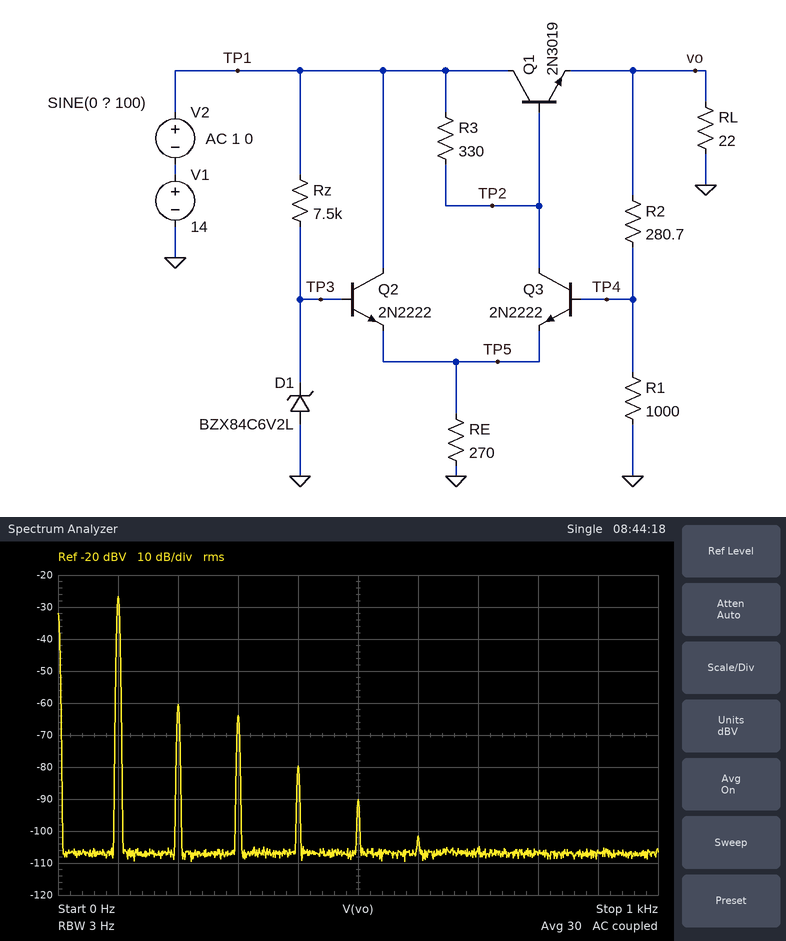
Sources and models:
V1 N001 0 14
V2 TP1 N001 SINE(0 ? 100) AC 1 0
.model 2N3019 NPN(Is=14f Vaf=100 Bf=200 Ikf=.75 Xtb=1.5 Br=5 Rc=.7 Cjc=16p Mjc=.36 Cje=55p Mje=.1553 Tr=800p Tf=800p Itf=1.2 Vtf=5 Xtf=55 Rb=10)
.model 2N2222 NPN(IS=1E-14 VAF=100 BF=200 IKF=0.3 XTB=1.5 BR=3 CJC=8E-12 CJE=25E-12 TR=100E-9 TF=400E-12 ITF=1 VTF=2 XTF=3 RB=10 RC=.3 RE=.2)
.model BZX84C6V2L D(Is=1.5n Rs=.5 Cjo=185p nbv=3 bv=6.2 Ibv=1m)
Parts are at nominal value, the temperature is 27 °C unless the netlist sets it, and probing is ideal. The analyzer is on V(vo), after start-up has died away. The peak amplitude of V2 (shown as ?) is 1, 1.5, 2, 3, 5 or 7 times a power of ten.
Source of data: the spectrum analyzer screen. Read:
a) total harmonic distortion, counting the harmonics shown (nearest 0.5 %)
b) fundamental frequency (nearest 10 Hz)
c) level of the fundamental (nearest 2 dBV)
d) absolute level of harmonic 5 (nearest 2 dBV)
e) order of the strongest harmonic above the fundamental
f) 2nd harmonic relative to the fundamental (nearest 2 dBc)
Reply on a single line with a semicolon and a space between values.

2.5 %; 100 Hz; -26 dBV; -90 dBV; 2; -34 dBc
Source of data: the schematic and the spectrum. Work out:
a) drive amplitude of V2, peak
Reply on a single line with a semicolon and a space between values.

1.5 V
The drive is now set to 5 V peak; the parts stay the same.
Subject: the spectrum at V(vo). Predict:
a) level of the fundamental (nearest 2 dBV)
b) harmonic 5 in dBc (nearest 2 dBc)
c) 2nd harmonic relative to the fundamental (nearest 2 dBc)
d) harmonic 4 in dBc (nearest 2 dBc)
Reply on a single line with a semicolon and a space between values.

-6 dBV; -42 dBc; -10 dBc; -34 dBc
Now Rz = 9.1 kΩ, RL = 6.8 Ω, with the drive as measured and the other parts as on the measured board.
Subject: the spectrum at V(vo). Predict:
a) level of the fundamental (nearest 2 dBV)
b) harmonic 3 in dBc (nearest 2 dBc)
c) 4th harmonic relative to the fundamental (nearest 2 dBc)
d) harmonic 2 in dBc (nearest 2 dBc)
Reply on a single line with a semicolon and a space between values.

-16 dBV; -14 dBc; -28 dBc; -8 dBc
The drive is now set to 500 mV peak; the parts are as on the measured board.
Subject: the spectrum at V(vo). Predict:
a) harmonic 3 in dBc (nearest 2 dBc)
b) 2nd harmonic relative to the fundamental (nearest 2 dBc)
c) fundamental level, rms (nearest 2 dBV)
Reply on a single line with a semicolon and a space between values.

-58 dBc; -46 dBc; -36 dBV
